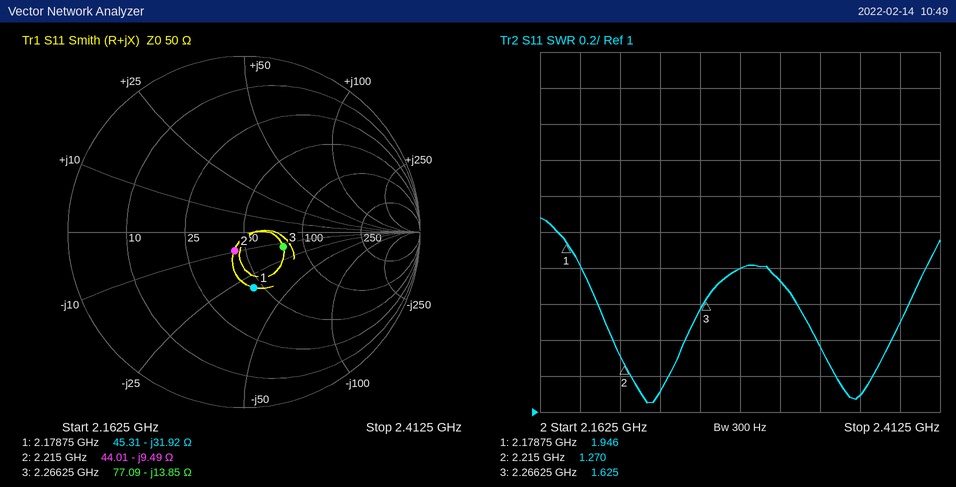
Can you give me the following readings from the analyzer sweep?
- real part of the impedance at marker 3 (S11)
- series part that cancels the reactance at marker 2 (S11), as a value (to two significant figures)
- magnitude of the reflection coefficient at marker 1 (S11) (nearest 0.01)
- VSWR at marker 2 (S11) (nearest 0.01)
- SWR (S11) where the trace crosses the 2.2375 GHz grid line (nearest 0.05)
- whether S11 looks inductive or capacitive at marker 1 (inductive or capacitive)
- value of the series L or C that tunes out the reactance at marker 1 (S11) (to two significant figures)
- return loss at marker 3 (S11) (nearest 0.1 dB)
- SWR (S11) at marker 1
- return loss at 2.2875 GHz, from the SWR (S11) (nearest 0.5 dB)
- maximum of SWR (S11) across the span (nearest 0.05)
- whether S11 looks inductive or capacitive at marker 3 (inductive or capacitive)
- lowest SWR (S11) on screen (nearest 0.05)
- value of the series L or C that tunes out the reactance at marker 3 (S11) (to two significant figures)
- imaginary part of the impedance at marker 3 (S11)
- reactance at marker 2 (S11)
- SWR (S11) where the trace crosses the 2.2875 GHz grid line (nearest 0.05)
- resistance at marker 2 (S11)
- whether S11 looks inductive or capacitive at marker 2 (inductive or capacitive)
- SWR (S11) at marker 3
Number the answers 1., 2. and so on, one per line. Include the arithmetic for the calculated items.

1. 77.09 Ω
2. L = 9.49 Ω/(2π × 2.215 GHz) ≈ 682 pH, so 680 pH to two significant figures
3. 0.32
4. 1.27
5. 1.10
6. capacitive
7. L = 31.92 Ω/(2π × 2.17875 GHz) ≈ 2.3 nH
8. 12.5 dB
9. 1.946
10. −20 log10((1.8 − 1)/(1.8 + 1)) ≈ 10.9 dB, so 11.0 dB to the nearest 0.5 dB
11. 2.10
12. capacitive
13. 1.05
14. L = 13.85 Ω/(2π × 2.26625 GHz) ≈ 973 pH, so 970 pH to two significant figures
15. -13.85 Ω
16. -9.49 Ω
17. 1.80
18. 44.01 Ω
19. capacitive
20. 1.625
